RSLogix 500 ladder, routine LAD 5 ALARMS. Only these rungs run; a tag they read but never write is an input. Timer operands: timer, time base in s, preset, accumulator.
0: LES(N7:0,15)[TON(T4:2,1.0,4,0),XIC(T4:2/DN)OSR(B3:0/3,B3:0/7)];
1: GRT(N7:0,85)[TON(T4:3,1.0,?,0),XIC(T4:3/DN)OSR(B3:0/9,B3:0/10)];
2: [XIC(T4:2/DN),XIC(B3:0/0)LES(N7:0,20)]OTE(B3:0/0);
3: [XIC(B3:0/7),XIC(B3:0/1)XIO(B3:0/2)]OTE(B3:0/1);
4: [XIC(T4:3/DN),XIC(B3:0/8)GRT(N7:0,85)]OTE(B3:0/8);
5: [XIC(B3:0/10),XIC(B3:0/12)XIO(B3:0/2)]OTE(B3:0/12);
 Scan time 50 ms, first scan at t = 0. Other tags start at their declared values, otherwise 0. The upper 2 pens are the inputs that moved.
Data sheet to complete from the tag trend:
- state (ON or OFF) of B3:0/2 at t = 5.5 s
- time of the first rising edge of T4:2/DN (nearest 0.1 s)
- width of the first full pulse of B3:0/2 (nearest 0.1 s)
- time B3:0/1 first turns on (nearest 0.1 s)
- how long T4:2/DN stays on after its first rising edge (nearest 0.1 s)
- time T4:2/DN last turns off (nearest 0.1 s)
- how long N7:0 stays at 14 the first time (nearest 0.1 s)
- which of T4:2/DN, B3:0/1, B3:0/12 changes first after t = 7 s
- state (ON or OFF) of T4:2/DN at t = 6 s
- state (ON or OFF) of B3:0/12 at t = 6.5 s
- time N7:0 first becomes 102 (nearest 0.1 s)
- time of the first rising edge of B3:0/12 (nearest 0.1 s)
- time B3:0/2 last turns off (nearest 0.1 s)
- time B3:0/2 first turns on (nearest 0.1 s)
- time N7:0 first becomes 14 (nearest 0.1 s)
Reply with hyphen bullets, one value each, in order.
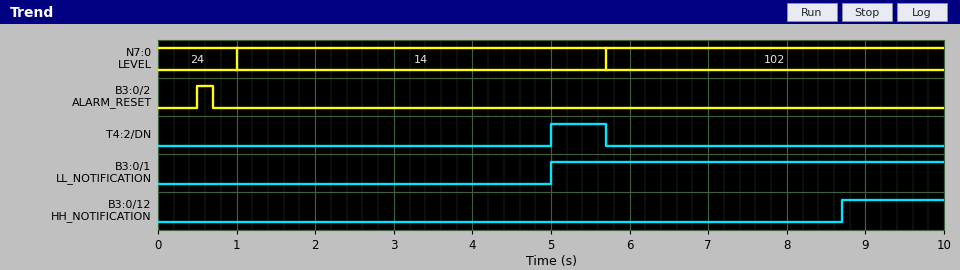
- OFF
- 5.0 s
- 0.2 s
- 5.0 s
- 0.7 s
- 5.7 s
- 4.7 s
- B3:0/12
- OFF
- OFF
- 5.7 s
- 8.7 s
- 0.7 s
- 0.5 s
- 1.0 s
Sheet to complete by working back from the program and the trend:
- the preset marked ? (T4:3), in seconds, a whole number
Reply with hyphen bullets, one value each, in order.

- 3 s
